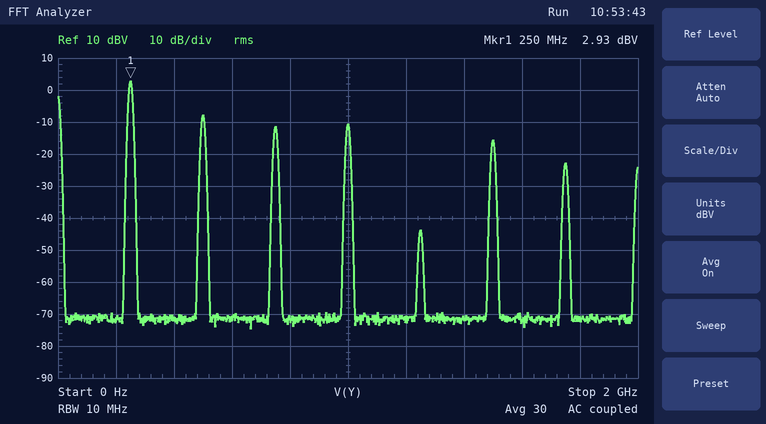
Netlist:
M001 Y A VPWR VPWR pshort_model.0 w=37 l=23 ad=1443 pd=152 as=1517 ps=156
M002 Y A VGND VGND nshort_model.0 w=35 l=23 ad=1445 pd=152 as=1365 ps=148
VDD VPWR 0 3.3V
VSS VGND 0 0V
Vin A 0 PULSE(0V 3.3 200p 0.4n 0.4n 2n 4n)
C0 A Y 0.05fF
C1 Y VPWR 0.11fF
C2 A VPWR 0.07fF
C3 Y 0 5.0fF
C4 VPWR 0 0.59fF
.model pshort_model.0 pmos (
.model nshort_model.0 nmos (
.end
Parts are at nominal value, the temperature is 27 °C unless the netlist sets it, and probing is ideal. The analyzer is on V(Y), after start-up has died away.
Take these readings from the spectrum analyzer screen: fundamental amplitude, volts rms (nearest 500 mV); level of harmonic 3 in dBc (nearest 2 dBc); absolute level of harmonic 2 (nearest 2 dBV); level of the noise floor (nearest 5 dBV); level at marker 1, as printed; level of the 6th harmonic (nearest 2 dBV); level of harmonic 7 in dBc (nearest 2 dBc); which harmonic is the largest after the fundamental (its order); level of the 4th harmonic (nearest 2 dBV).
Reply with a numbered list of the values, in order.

1. 1.5 V
2. -14 dBc
3. -8 dBV
4. -70 dBV
5. 2.93 dBV
6. -16 dBV
7. -26 dBc
8. 2
9. -10 dBV
